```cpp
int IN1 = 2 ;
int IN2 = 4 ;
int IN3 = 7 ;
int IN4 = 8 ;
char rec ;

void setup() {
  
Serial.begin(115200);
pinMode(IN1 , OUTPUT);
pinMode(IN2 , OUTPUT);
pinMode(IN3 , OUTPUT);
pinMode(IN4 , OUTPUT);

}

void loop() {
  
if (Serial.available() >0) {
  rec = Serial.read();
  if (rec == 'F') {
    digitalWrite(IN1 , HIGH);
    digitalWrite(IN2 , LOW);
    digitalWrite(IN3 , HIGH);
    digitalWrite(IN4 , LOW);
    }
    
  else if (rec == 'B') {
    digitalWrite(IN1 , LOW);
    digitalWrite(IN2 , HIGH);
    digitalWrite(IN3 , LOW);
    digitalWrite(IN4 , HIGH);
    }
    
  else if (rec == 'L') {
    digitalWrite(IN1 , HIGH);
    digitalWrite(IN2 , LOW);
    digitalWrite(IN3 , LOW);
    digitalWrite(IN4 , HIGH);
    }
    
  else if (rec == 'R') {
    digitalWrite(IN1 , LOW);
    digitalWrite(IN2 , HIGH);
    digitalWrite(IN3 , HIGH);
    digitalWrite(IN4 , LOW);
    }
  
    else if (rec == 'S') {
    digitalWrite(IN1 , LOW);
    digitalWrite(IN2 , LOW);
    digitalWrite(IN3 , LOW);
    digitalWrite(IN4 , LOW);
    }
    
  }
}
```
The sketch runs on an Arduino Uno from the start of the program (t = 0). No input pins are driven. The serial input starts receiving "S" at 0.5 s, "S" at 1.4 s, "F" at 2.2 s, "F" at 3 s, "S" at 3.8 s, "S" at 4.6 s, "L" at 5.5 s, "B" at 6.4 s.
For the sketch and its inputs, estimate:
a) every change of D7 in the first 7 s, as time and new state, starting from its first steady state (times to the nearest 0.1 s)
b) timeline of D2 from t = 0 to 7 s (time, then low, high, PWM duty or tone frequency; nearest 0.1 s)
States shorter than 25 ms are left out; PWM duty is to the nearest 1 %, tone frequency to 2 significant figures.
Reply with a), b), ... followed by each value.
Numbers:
a) 0 s low; 2.2 s high; 3.8 s low
b) 0 s low; 2.2 s high; 3.8 s low; 5.5 s high; 6.4 s low
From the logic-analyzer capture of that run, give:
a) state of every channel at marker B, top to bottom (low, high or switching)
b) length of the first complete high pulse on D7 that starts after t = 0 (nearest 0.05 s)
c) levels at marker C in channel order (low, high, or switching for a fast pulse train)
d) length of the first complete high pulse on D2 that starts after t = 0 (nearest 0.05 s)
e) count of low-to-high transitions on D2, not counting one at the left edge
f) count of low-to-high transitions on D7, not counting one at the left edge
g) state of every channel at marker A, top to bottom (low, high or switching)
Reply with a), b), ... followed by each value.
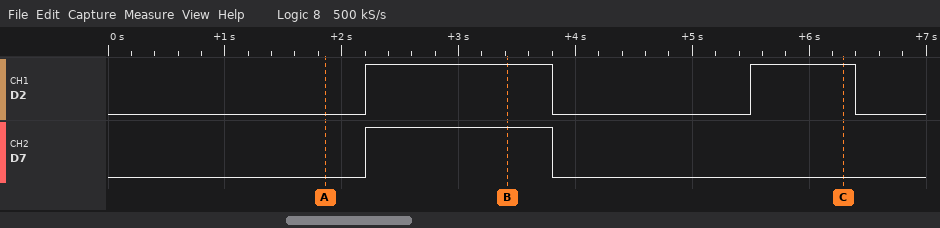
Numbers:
a) D2 high, D7 high
b) 1.60 s
c) D2 high, D7 low
d) 1.60 s
e) 2
f) 1
g) D2 low, D7 low
